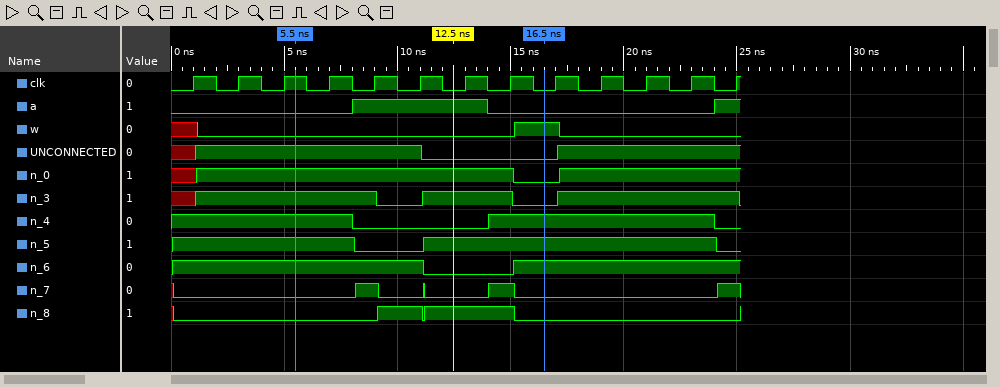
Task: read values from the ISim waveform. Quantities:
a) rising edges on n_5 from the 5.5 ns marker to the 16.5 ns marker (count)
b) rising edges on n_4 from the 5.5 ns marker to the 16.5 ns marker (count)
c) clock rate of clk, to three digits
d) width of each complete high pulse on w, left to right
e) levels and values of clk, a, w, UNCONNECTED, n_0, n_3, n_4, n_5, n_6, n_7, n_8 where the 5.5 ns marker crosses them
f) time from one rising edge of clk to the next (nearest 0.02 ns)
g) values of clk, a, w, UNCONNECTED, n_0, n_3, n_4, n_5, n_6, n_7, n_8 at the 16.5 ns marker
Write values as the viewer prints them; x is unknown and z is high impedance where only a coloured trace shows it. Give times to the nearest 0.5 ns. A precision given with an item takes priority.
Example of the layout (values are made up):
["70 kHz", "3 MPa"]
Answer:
["1", "1", "500 MHz", "2 ns", "clk=1, a=0, w=0, UNCONNECTED=1, n_0=1, n_3=1, n_4=1, n_5=1, n_6=1, n_7=0, n_8=0", "2 ns", "clk=0, a=0, w=1, UNCONNECTED=0, n_0=0, n_3=0, n_4=1, n_5=1, n_6=1, n_7=0, n_8=0"]
